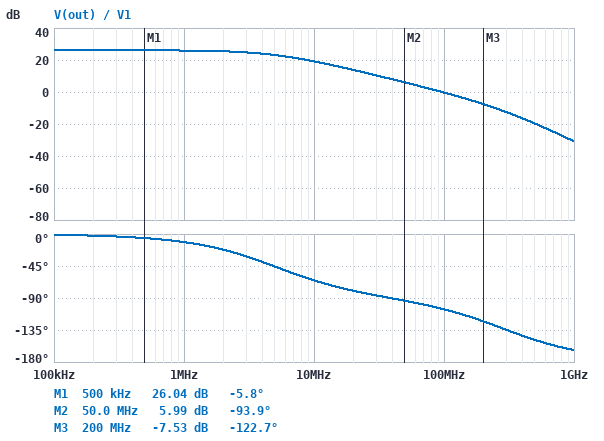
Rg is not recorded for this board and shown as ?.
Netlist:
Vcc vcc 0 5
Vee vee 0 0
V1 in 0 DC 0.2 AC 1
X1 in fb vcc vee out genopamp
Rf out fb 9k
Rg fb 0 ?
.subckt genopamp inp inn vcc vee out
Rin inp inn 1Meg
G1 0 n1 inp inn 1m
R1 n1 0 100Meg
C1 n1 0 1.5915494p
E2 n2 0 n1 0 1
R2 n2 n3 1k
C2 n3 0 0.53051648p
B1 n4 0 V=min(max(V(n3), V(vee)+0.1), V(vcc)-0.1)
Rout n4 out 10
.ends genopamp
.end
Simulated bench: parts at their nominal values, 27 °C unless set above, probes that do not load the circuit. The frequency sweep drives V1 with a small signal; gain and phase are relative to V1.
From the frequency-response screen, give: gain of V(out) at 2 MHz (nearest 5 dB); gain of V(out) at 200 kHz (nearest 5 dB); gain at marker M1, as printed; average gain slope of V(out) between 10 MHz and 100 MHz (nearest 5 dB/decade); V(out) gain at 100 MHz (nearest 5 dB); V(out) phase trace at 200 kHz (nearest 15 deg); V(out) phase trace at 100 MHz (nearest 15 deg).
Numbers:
25 dB
25 dB
26.04 dB
-20 dB/decade
0 dB
0 deg
-105 deg
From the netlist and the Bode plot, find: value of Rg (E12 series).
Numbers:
470 Ω
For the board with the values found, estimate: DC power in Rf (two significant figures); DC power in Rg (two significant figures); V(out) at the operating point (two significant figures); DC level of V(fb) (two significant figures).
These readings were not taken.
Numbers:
1.6 mW
85 µW
4.0 V
200 mV
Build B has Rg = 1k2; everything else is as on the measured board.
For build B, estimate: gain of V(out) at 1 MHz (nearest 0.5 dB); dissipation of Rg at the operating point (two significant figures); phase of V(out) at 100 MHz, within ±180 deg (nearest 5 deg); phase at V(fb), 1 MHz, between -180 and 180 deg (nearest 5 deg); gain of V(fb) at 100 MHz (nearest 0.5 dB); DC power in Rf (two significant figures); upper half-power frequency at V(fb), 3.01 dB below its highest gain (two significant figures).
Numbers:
18.5 dB
33 µW
-100 deg
-5 deg
-19.0 dB
250 µW
12 MHz
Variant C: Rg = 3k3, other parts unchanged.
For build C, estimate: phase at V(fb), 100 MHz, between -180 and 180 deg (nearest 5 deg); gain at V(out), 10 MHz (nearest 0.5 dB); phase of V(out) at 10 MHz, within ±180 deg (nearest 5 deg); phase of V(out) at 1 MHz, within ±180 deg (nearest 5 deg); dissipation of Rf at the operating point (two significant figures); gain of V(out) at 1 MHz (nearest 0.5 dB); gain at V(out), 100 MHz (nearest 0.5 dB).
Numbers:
-95 deg
11.0 dB
-20 deg
0 deg
33 µW
11.5 dB
0 dB
